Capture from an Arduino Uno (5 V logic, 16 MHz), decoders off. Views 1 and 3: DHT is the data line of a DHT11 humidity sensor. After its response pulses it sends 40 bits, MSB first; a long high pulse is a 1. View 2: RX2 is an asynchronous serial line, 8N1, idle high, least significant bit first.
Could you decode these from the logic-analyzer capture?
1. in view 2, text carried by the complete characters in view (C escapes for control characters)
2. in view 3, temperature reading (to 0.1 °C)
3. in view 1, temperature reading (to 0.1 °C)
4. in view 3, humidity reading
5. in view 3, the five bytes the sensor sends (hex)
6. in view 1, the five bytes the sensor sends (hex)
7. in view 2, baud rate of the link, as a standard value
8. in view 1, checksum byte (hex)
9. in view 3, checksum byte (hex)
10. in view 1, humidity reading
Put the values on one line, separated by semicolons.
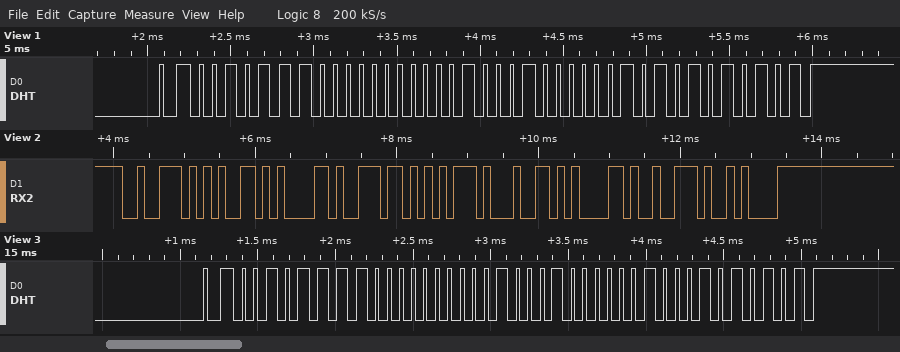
"reanudar\n"; 34.4 °C; 34.5 °C; 47 %; 2F 00 22 04 55; 2E 00 22 05 55; 9600 baud; 0x55; 0x55; 46 %
